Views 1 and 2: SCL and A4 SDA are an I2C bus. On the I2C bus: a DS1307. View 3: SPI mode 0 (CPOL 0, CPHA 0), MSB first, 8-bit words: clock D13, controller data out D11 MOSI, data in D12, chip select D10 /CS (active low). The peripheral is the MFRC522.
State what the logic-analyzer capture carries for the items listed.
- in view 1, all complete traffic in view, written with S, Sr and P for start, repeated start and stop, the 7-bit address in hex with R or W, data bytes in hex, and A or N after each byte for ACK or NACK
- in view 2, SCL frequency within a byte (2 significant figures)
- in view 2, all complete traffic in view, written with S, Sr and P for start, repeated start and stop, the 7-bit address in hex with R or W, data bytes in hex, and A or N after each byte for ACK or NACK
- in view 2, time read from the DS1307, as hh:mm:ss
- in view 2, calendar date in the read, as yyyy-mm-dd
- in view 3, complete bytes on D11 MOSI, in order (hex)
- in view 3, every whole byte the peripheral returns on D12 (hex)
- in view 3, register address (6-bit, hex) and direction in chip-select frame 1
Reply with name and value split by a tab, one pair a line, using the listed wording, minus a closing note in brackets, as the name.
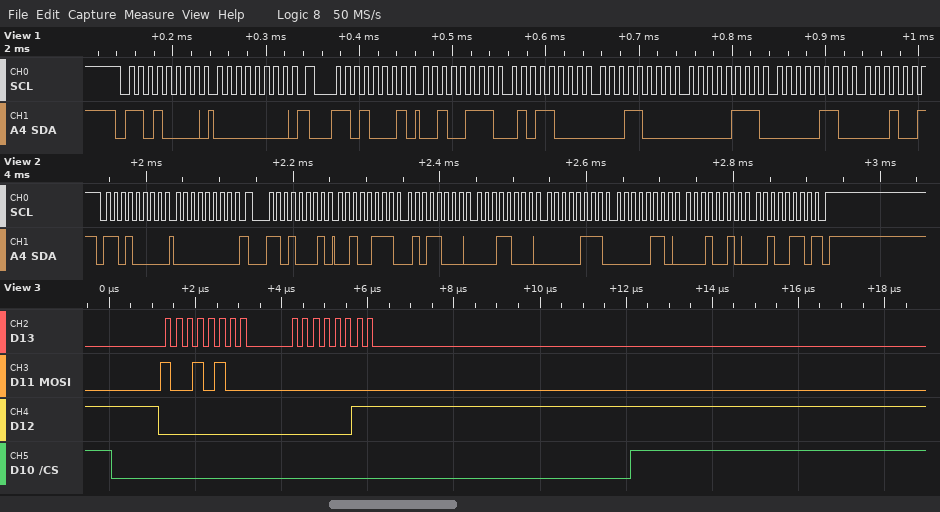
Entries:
in view 1, all complete traffic in view, written with S, Sr and P for start, repeated start and stop, the 7-bit address in hex with R or W, data bytes in hex, and A or N after each byte for ACK or NACK	S 68W A 00 A Sr 68R A 27 A 58 A 18 A 07 A 06 A
in view 2, SCL frequency within a byte	100 kHz
in view 2, all complete traffic in view, written with S, Sr and P for start, repeated start and stop, the 7-bit address in hex with R or W, data bytes in hex, and A or N after each byte for ACK or NACK	S 68W A 00 A Sr 68R A 27 A 58 A 18 A 07 A 06 A 12 A 26 N P
in view 2, time read from the DS1307, as hh:mm:ss	18:58:27
in view 2, calendar date in the read, as yyyy-mm-dd	2026-12-06
in view 3, complete bytes on D11 MOSI, in order	94 00
in view 3, every whole byte the peripheral returns on D12	00 03
in view 3, register address (6-bit, hex) and direction in chip-select frame 1	0x0A read
